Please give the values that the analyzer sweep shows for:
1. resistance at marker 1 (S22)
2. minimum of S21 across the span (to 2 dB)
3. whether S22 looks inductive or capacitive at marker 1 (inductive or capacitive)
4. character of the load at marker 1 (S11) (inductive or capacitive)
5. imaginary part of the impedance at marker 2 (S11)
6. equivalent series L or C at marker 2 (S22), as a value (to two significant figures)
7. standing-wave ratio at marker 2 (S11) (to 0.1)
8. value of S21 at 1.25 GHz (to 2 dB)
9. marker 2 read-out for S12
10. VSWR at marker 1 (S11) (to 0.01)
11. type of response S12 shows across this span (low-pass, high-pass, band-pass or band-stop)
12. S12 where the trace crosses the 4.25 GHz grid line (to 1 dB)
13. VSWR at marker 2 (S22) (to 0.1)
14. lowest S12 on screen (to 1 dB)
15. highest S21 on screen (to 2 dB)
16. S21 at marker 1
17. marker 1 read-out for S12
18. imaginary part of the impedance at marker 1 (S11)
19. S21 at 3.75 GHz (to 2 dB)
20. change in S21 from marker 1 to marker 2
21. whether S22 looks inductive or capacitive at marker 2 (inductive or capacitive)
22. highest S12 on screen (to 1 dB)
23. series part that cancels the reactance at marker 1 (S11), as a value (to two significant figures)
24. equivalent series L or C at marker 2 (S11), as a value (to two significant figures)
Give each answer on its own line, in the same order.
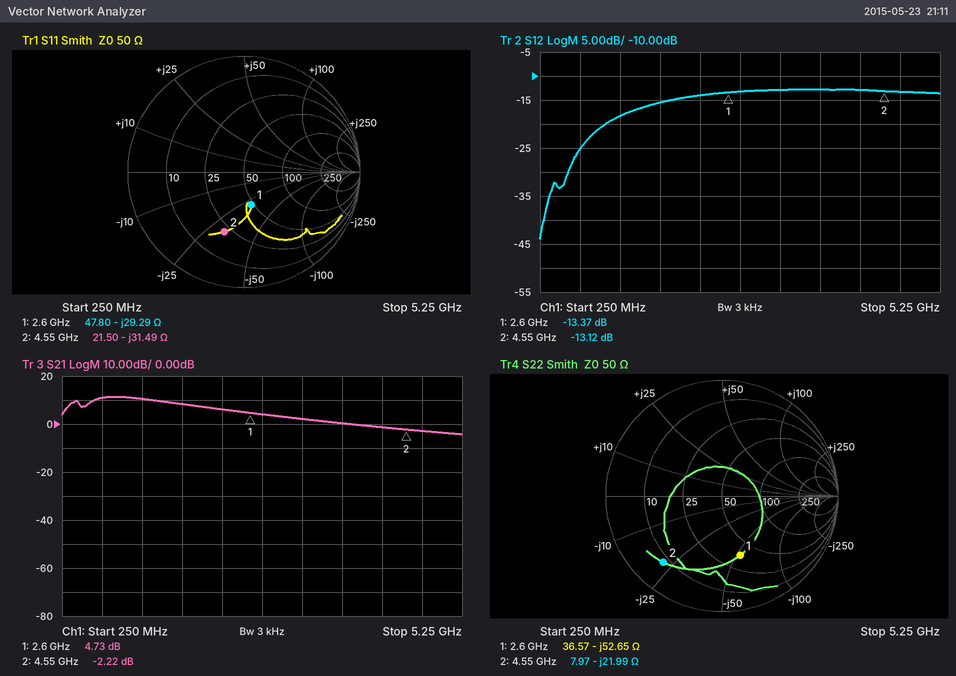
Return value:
36.57 Ω
-4 dB
capacitive
capacitive
-31.49 Ω
1.6 pF
3.4
10 dB
-13.12 dB
1.81
high-pass
-13 dB
7.5
-44 dB
12 dB
4.73 dB
-13.37 dB
-29.29 Ω
0 dB
-6.95 dB
capacitive
-13 dB
1.8 nH
1.1 pF
